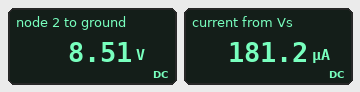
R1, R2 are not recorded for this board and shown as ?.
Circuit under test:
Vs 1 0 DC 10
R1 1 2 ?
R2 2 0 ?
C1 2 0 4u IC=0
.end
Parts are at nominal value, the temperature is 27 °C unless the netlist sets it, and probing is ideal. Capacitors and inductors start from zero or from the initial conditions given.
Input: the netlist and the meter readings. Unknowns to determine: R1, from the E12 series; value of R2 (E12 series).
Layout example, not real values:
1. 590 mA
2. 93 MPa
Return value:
1. 8.2 kΩ
2. 47 kΩ
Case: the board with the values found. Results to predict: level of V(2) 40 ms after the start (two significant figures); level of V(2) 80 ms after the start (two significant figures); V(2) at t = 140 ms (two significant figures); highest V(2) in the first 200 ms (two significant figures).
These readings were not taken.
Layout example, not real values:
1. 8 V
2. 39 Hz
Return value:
1. 6.5 V
2. 8.0 V
3. 8.5 V
4. 8.5 V
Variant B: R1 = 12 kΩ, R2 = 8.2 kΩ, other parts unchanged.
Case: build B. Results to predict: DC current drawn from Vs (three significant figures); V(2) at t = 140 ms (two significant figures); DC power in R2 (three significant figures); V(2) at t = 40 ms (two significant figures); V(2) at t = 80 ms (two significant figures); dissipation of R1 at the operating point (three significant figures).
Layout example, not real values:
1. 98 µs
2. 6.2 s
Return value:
1. 495 µA
2. 4.1 V
3. 2.01 mW
4. 3.5 V
5. 4.0 V
6. 2.94 mW
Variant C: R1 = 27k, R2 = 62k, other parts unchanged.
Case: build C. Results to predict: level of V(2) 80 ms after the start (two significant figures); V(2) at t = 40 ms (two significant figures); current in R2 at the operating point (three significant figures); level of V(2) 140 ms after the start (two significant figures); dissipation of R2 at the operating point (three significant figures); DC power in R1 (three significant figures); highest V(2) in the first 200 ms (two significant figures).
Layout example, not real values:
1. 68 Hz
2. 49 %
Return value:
1. 4.6 V
2. 2.9 V
3. 112 µA
4. 5.9 V
5. 783 µW
6. 341 µW
7. 6.5 V
